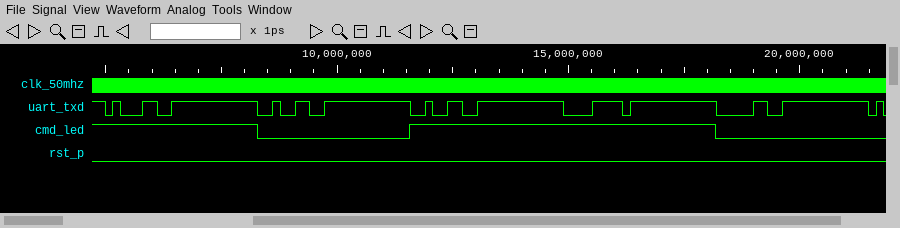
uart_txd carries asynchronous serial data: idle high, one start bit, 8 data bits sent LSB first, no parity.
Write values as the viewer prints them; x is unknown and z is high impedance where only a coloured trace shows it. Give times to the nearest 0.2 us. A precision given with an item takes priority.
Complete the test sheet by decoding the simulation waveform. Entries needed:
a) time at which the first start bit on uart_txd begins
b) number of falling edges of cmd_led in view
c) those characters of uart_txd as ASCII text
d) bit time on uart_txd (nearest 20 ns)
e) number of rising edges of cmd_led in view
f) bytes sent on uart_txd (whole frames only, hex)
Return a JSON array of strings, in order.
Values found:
["5 us", "2", "\"122x0\"", "160 ns", "1", "31, 32, 32, 78, 30"]
